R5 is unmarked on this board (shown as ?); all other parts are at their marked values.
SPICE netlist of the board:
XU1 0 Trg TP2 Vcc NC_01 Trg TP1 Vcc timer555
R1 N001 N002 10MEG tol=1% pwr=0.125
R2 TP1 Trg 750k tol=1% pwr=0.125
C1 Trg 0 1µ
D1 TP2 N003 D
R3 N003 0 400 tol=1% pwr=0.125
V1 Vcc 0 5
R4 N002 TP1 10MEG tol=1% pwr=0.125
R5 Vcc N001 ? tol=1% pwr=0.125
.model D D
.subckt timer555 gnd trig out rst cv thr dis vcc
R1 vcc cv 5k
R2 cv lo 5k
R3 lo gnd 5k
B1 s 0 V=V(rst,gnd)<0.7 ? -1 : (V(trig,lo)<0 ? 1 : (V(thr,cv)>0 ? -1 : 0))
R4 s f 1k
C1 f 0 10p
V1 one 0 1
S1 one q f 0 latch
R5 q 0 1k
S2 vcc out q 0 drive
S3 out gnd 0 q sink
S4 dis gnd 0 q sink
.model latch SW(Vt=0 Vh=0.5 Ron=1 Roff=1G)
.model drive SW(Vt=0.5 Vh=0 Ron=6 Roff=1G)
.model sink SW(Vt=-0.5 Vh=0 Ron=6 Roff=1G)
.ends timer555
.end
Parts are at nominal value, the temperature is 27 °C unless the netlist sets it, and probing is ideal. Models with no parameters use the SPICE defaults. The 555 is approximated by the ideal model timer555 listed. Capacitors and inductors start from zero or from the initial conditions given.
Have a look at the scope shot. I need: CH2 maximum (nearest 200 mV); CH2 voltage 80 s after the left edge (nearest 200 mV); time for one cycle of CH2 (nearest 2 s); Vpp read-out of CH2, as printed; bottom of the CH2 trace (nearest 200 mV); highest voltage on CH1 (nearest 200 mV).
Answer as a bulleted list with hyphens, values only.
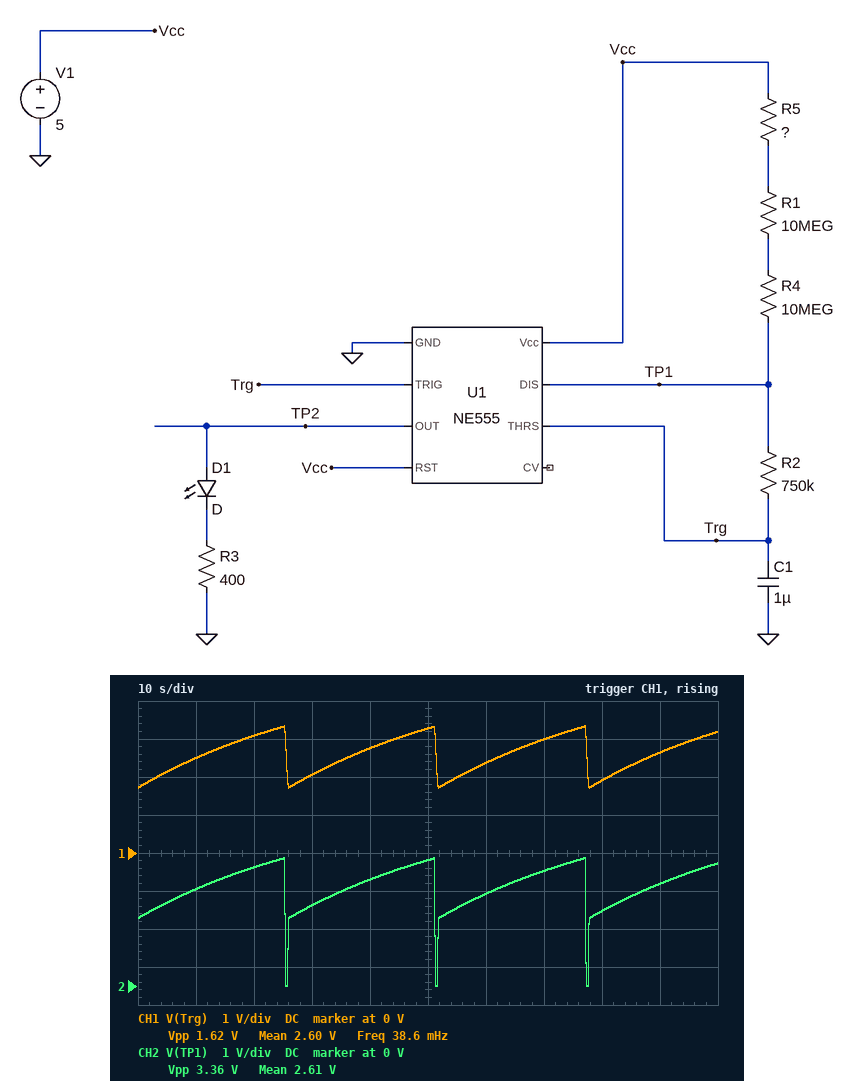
- 3.4 V
- 2.0 V
- 26 s
- 3.36 V
- 0 V
- 3.4 V
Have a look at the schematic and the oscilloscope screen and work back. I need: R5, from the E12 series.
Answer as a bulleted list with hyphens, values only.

- 15 MΩ
